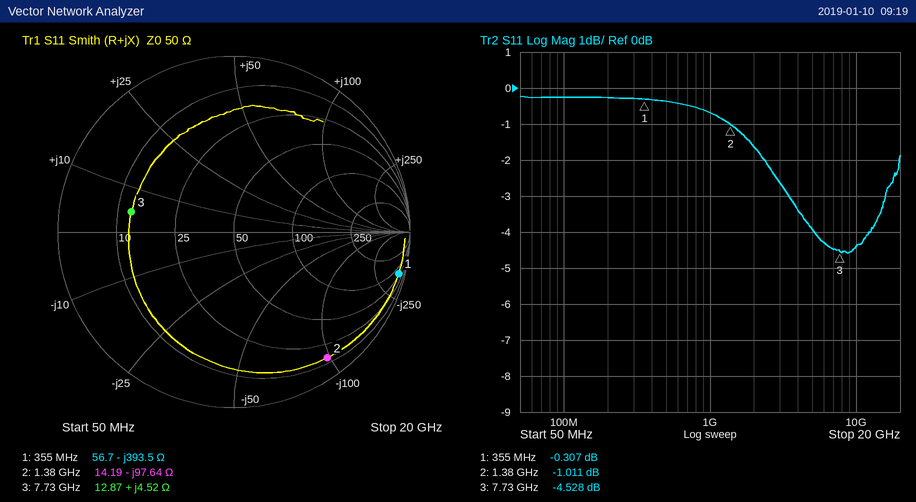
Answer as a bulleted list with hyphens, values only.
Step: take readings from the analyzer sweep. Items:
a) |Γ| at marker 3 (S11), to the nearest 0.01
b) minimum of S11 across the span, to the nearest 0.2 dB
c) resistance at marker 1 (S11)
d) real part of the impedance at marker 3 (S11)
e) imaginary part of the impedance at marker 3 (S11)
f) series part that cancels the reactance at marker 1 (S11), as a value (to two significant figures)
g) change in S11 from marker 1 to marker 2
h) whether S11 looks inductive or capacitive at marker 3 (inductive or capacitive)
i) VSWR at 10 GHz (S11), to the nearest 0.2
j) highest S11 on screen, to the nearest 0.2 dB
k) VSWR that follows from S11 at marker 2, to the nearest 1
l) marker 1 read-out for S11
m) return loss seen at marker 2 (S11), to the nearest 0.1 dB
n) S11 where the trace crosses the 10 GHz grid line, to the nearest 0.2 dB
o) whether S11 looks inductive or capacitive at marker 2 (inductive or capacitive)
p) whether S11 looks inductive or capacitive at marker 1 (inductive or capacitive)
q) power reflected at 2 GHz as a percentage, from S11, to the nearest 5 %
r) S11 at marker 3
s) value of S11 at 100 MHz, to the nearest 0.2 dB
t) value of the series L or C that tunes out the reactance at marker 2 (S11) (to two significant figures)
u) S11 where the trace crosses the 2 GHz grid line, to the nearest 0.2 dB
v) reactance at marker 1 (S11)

- 0.59
- -4.6 dB
- 56.7 Ω
- 12.87 Ω
- +4.52 Ω
- 180 nH
- -0.704 dB
- inductive
- 4.0
- -0.2 dB
- 17
- -0.307 dB
- 1.0 dB
- -4.4 dB
- capacitive
- capacitive
- 70 %
- -4.528 dB
- -0.2 dB
- 11 nH
- -1.6 dB
- -393.5 Ω
